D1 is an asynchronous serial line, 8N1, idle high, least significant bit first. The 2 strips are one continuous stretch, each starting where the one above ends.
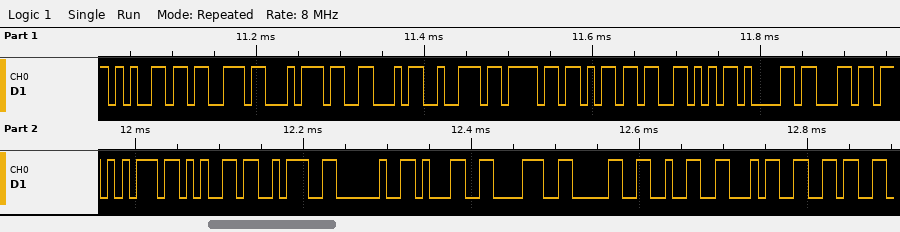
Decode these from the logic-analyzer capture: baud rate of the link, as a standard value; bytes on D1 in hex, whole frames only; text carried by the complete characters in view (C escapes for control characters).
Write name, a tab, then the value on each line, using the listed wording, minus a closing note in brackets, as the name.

baud rate of the link, as a standard value	115200 baud
bytes on D1 in hex, whole frames only	65 73 74 46 72 6F 6D 56 61 6C 75 65 3A 20 31 38 30 32 34 36
text carried by the complete characters in view	"estFromValue: 180246"
